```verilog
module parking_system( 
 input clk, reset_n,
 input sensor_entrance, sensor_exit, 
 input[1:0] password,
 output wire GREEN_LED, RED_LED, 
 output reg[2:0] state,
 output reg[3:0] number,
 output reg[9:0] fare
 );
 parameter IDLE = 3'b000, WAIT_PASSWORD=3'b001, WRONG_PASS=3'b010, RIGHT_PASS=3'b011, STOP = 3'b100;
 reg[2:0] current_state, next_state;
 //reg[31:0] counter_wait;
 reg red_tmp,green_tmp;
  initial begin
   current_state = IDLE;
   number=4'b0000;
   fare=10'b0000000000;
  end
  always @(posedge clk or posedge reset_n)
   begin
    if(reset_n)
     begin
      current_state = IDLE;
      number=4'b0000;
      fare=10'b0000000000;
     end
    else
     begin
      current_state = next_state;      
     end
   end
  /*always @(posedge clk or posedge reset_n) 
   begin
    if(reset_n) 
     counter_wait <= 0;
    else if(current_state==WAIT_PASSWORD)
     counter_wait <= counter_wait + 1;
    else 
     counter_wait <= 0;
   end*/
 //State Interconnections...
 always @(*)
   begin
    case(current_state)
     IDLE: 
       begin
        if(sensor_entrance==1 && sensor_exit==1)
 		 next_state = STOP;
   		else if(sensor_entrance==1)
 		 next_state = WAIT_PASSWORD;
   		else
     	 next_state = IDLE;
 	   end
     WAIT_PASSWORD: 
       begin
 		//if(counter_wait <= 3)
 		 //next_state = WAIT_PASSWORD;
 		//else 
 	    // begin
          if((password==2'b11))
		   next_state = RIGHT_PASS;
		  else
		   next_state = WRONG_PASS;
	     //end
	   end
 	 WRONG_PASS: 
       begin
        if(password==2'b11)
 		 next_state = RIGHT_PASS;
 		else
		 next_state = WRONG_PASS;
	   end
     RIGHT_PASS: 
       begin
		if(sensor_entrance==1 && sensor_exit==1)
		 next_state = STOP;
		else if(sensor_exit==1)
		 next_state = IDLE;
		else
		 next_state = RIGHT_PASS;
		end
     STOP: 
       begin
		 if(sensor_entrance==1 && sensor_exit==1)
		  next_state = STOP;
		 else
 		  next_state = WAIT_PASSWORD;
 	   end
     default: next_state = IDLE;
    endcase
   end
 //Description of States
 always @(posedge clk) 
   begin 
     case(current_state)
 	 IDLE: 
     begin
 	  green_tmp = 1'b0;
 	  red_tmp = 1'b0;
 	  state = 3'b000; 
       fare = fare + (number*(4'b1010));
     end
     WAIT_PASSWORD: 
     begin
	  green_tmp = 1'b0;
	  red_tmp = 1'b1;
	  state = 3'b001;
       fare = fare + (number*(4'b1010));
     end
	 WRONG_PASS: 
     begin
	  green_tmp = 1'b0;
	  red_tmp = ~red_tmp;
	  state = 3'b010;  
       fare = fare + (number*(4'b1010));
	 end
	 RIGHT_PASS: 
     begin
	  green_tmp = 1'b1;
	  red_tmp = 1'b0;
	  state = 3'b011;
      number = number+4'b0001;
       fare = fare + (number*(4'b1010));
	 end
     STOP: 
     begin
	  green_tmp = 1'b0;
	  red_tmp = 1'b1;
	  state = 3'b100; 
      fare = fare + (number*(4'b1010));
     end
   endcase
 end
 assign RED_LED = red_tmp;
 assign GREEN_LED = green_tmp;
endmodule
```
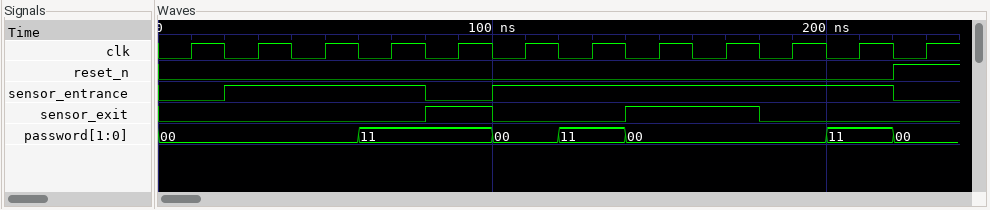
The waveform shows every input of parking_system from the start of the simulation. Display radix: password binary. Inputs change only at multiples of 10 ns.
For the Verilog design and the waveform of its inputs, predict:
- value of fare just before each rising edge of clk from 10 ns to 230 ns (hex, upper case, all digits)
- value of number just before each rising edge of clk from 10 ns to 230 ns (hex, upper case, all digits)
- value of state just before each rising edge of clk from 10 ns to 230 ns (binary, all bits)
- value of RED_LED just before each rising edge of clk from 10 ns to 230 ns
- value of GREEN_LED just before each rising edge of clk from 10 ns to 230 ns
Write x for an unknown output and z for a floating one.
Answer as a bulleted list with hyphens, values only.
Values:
- 000, 000, 000, 000, 00A, 014, 01E, 032, 046, 05A, 06E, 000
- 0, 0, 0, 0, 1, 1, 1, 2, 2, 2, 2, 0
- x, 000, 001, 010, 011, 000, 001, 011, 100, 100, 001, 011
- x 0 1 0 0 0 1 0 1 1 1 0
- x 0 0 0 1 0 0 1 0 0 0 1
